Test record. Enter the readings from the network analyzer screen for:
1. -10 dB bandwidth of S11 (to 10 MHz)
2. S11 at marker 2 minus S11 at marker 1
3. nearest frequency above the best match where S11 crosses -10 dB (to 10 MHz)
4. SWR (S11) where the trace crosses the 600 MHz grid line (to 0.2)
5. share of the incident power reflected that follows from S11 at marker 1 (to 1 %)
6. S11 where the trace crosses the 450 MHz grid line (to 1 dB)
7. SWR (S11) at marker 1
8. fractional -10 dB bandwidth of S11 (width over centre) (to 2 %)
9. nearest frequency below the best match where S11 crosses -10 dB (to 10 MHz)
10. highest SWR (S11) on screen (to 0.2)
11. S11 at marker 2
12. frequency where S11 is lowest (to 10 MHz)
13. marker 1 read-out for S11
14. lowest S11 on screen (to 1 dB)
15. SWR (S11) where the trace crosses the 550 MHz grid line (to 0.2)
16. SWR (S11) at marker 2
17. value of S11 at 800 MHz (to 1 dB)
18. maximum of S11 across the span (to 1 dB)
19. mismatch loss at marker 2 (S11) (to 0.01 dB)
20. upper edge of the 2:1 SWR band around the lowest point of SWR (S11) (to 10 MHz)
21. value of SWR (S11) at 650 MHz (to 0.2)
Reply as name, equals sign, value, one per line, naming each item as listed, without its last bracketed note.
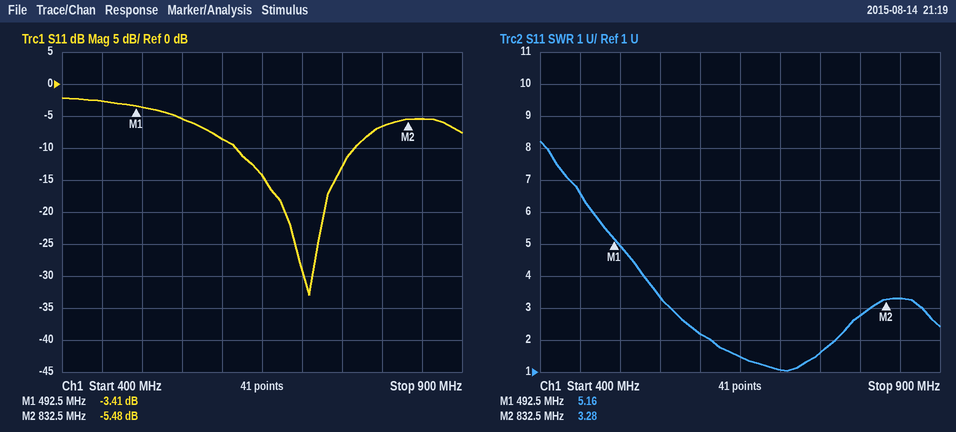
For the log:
-10 dB bandwidth of S11 = 150 MHz
S11 at marker 2 minus S11 at marker 1 = -2.07 dB
nearest frequency above the best match where S11 crosses -10 dB = 770 MHz
SWR (S11) where the trace crosses the 600 MHz grid line = 2.2
share of the incident power reflected that follows from S11 at marker 1 = 46 %
S11 where the trace crosses the 450 MHz grid line = -3 dB
SWR (S11) at marker 1 = 5.16
fractional -10 dB bandwidth of S11 (width over centre) = 22 %
nearest frequency below the best match where S11 crosses -10 dB = 620 MHz
highest SWR (S11) on screen = 8.2
S11 at marker 2 = -5.48 dB
frequency where S11 is lowest = 710 MHz
marker 1 read-out for S11 = -3.41 dB
lowest S11 on screen = -33 dB
SWR (S11) where the trace crosses the 550 MHz grid line = 3.4
SWR (S11) at marker 2 = 3.28
value of S11 at 800 MHz = -7 dB
maximum of S11 across the span = -2 dB
mismatch loss at marker 2 (S11) = 1.45 dB
upper edge of the 2:1 SWR band around the lowest point of SWR (S11) = 770 MHz
value of SWR (S11) at 650 MHz = 1.4
